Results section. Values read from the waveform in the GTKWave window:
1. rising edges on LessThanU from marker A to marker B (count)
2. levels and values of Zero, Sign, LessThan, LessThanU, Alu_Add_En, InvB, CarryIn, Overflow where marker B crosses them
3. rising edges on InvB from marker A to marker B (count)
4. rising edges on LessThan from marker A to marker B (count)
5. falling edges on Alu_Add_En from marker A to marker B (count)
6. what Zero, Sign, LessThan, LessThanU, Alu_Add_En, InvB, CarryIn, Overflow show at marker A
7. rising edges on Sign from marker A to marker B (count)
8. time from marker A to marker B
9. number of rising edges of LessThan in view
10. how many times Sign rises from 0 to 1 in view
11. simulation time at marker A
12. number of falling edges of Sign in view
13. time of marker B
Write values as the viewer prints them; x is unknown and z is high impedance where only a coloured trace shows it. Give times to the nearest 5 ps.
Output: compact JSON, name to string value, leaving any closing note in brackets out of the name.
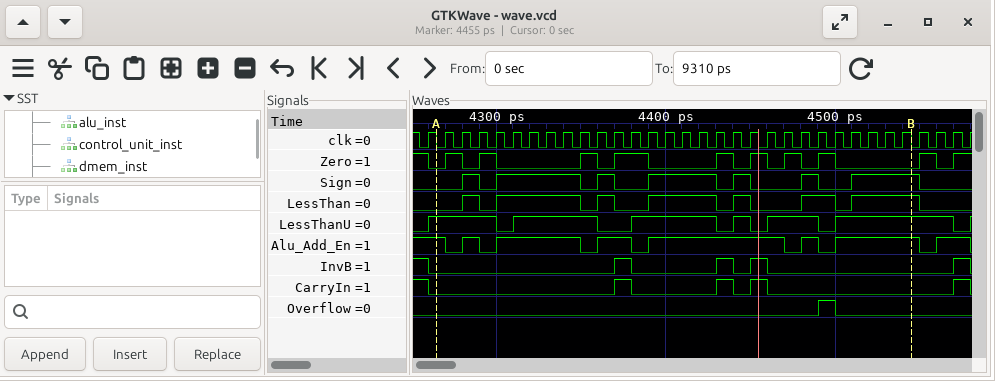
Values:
{"rising edges on LessThanU from marker A to marker B": "5", "levels and values of Zero, Sign, LessThan, LessThanU, Alu_Add_En, InvB, CarryIn, Overflow where marker B crosses them": "Zero=0, Sign=1, LessThan=1, LessThanU=1, Alu_Add_En=1, InvB=0, CarryIn=0, Overflow=0", "rising edges on InvB from marker A to marker B": "3", "rising edges on LessThan from marker A to marker B": "7", "falling edges on Alu_Add_En from marker A to marker B": "6", "what Zero, Sign, LessThan, LessThanU, Alu_Add_En, InvB, CarryIn, Overflow show at marker A": "Zero=0, Sign=0, LessThan=0, LessThanU=1, Alu_Add_En=1, InvB=0, CarryIn=0, Overflow=0", "rising edges on Sign from marker A to marker B": "7", "time from marker A to marker B": "280 ps", "number of rising edges of LessThan in view": "7", "how many times Sign rises from 0 to 1 in view": "7", "simulation time at marker A": "4265 ps", "number of falling edges of Sign in view": "7", "time of marker B": "4545 ps"}
